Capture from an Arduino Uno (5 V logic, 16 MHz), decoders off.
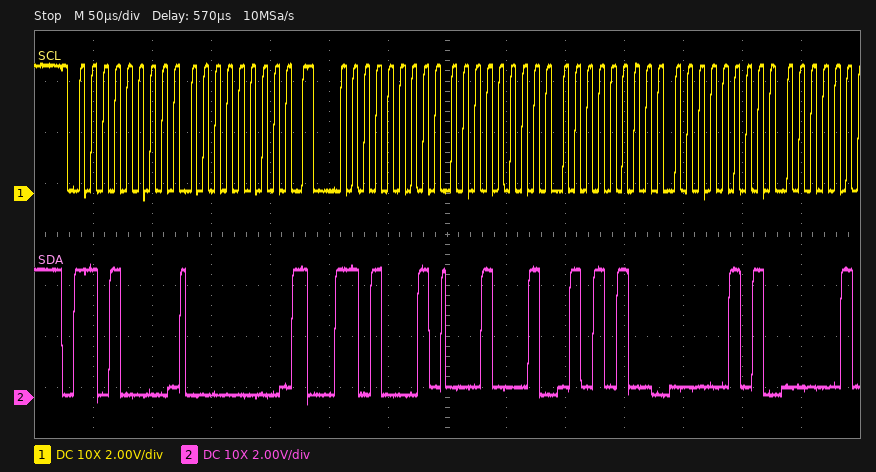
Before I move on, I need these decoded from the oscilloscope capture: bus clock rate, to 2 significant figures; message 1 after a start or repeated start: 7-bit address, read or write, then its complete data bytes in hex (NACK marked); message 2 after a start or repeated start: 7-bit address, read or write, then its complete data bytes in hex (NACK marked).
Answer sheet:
100 kHz
0x68 write: 00
0x68 read: 11 54 05
